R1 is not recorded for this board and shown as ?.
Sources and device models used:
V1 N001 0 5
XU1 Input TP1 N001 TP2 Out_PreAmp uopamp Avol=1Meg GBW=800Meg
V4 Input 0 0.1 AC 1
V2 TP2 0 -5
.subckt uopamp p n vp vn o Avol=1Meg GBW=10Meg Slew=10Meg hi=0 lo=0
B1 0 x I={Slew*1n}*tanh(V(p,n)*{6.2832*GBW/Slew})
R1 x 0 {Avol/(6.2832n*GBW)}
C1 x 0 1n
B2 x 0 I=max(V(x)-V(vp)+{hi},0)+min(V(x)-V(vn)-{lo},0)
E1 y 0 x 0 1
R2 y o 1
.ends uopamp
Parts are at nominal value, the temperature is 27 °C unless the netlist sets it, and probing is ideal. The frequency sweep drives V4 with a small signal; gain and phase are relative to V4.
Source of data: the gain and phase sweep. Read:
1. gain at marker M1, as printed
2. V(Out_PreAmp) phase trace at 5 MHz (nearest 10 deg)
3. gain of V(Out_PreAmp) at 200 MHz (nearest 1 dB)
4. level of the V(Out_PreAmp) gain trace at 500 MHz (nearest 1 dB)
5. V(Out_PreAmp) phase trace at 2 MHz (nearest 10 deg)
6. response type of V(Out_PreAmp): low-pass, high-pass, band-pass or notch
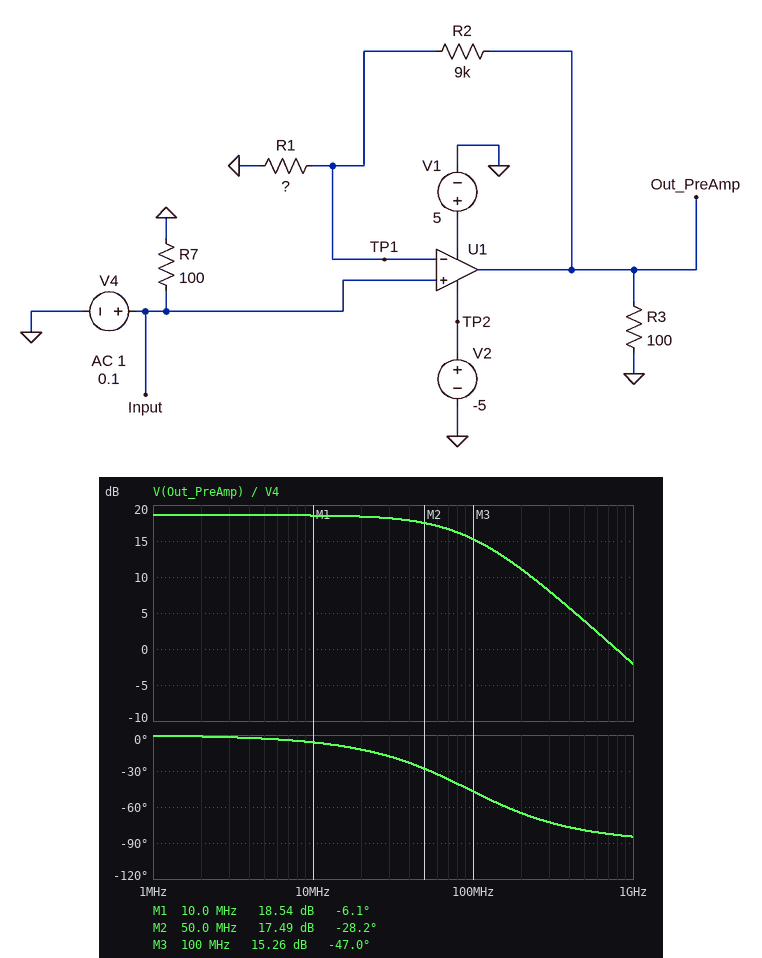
18.54 dB
0 deg
11 dB
4 dB
0 deg
low-pass
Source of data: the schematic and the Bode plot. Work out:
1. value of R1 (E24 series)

1.2 kΩ
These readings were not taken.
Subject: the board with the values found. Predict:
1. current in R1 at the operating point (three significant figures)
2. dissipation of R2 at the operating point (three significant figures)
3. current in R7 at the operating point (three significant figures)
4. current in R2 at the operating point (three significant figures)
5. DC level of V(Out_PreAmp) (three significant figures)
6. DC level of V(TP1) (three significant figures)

83.3 µA
62.5 µW
1.00 mA
83.3 µA
850 mV
100 mV
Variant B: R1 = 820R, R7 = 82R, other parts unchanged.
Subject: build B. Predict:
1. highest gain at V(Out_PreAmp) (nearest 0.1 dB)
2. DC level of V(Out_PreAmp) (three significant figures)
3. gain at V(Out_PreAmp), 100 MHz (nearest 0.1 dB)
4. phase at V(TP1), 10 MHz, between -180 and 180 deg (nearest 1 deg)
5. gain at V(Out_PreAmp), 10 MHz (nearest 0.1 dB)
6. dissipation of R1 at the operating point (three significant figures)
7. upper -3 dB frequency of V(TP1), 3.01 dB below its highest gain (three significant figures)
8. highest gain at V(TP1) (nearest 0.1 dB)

21.6 dB
1.20 V
16.4 dB
-9 deg
21.5 dB
12.2 µW
66.1 MHz
0 dB
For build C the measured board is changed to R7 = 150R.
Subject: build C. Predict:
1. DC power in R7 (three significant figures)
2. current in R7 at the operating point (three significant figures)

66.7 µW
667 µA
